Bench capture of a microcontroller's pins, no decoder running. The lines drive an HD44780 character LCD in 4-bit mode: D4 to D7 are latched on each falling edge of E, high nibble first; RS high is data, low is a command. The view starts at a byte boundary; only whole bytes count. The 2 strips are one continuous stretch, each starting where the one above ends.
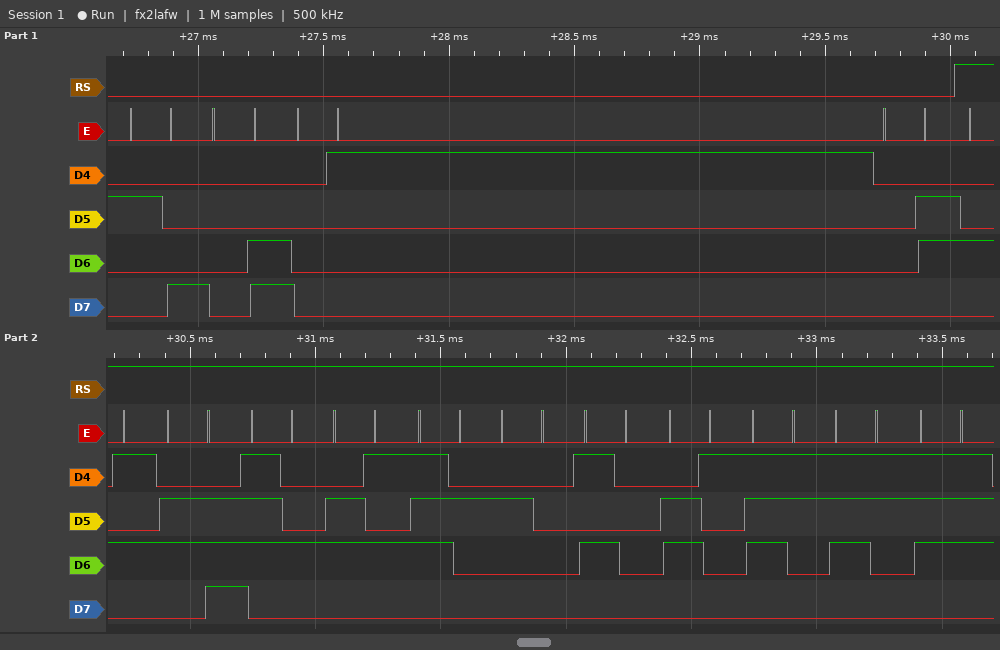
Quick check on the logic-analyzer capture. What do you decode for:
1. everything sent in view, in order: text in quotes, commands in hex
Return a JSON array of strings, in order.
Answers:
["0x28 0x0C 0x01 0x06 \"Enter Passw\""]
